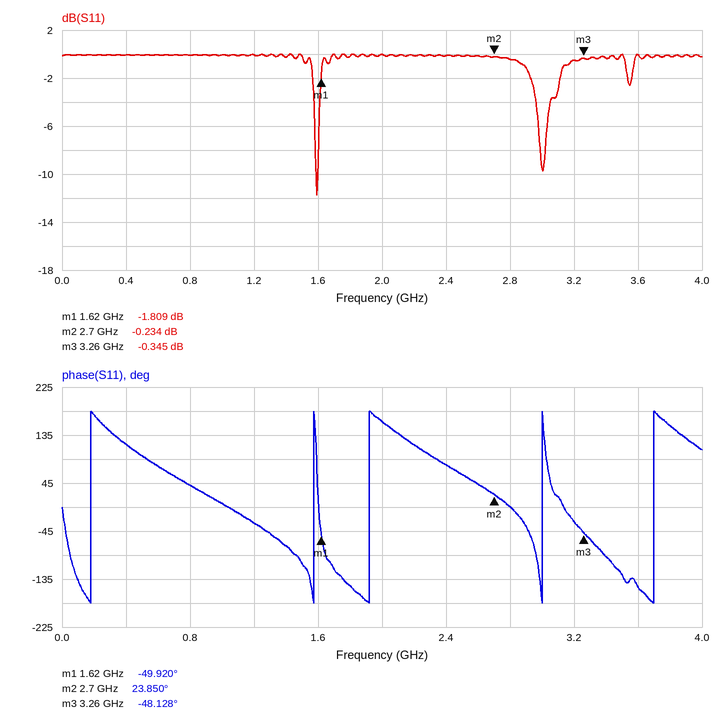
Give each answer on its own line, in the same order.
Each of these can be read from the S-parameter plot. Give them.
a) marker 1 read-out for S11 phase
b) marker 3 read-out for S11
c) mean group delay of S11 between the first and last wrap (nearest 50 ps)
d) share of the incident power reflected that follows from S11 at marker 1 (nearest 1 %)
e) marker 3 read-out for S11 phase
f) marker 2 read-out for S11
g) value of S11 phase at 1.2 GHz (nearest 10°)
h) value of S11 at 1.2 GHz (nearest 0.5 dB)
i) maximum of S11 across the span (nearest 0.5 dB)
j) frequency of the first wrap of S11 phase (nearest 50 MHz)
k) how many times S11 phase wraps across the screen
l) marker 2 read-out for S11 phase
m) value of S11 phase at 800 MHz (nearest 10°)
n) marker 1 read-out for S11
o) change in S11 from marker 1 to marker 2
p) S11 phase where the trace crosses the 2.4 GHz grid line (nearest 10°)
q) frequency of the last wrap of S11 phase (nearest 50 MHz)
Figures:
-49.920°
-0.345 dB
1.15 ns
66 %
-48.128°
-0.234 dB
-30°
0.0 dB
0.0 dB
200 MHz
5
23.850°
40°
-1.809 dB
1.575 dB
80°
3.70 GHz
